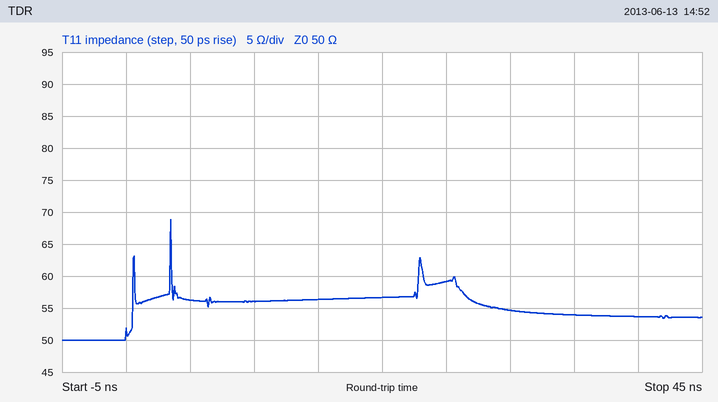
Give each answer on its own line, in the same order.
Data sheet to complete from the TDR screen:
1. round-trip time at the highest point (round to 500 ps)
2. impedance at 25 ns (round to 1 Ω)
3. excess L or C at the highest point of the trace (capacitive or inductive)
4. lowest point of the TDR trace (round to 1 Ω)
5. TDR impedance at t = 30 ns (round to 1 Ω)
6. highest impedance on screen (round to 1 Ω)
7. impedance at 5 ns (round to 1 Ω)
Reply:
3.5 ns
59 Ω
inductive
50 Ω
55 Ω
69 Ω
56 Ω
